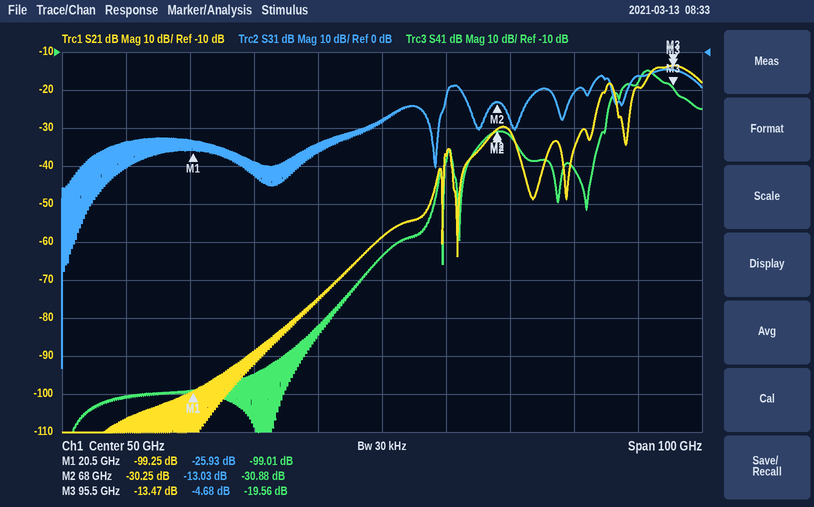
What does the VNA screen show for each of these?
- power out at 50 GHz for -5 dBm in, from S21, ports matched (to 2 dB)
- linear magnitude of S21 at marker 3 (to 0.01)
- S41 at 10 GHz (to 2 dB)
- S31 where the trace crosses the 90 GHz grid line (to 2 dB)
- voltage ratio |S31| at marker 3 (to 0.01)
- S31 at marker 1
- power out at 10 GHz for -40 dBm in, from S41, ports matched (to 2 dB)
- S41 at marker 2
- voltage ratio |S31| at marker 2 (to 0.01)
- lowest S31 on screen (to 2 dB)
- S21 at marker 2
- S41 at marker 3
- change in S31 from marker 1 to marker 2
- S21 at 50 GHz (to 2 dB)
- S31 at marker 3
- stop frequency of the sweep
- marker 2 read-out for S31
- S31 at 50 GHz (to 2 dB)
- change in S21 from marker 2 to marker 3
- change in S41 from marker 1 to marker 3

-64 dBm
0.21
-100 dB
-6 dB
0.58
-25.93 dB
-140 dBm
-30.88 dB
0.22
-84 dB
-30.25 dB
-19.56 dB
12.90 dB
-58 dB
-4.68 dB
100 GHz
-13.03 dB
-18 dB
16.78 dB
79.45 dB
